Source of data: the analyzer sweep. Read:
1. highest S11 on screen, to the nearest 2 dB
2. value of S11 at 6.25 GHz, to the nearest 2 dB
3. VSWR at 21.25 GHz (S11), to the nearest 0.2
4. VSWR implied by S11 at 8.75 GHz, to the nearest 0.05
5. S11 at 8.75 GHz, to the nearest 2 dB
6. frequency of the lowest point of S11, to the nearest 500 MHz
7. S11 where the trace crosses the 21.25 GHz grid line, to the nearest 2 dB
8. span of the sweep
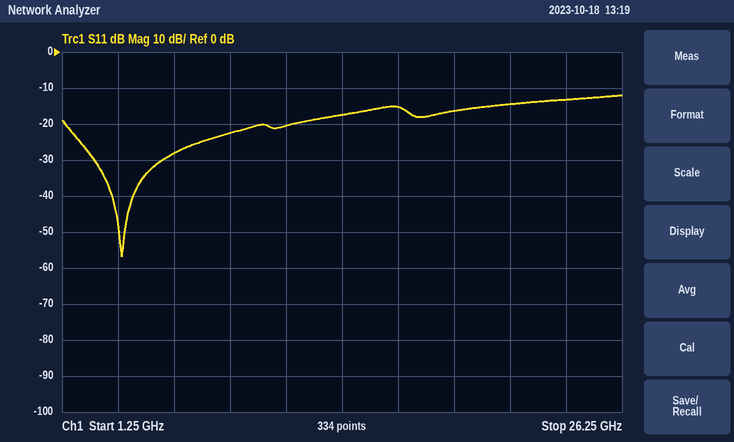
-12 dB
-28 dB
1.4
1.15
-22 dB
4.0 GHz
-14 dB
25 GHz
